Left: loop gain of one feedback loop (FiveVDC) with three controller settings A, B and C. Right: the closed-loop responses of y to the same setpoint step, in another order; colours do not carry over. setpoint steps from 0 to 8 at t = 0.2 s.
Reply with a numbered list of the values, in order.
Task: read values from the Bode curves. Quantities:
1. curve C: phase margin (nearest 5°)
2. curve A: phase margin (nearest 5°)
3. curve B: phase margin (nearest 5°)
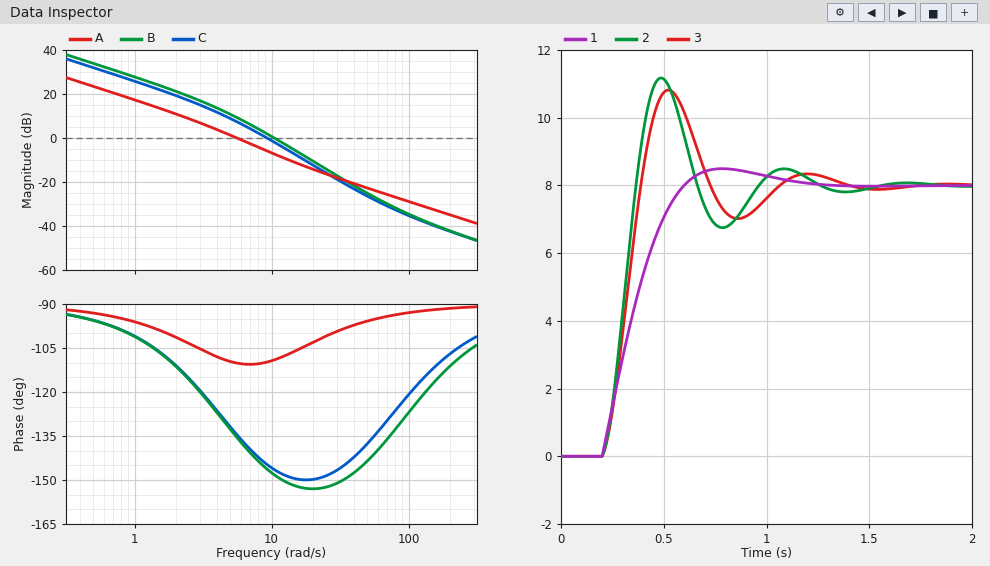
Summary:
1. 35°
2. 70°
3. 30°
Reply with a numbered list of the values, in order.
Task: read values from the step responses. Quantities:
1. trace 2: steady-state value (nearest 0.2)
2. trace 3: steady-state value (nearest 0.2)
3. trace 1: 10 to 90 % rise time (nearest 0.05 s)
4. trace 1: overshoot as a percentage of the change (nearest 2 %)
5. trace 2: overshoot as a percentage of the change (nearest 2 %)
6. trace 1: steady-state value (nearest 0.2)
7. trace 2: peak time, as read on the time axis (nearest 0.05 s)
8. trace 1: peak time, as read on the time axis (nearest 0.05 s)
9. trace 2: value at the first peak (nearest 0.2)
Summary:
1. 8.0
2. 8.0
3. 0.30 s
4. 6 %
5. 40 %
6. 8.0
7. 0.50 s
8. 0.80 s
9. 11.2
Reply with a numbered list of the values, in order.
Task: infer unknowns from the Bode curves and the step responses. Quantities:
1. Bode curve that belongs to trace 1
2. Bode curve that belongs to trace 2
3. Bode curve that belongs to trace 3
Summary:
1. A
2. B
3. C
